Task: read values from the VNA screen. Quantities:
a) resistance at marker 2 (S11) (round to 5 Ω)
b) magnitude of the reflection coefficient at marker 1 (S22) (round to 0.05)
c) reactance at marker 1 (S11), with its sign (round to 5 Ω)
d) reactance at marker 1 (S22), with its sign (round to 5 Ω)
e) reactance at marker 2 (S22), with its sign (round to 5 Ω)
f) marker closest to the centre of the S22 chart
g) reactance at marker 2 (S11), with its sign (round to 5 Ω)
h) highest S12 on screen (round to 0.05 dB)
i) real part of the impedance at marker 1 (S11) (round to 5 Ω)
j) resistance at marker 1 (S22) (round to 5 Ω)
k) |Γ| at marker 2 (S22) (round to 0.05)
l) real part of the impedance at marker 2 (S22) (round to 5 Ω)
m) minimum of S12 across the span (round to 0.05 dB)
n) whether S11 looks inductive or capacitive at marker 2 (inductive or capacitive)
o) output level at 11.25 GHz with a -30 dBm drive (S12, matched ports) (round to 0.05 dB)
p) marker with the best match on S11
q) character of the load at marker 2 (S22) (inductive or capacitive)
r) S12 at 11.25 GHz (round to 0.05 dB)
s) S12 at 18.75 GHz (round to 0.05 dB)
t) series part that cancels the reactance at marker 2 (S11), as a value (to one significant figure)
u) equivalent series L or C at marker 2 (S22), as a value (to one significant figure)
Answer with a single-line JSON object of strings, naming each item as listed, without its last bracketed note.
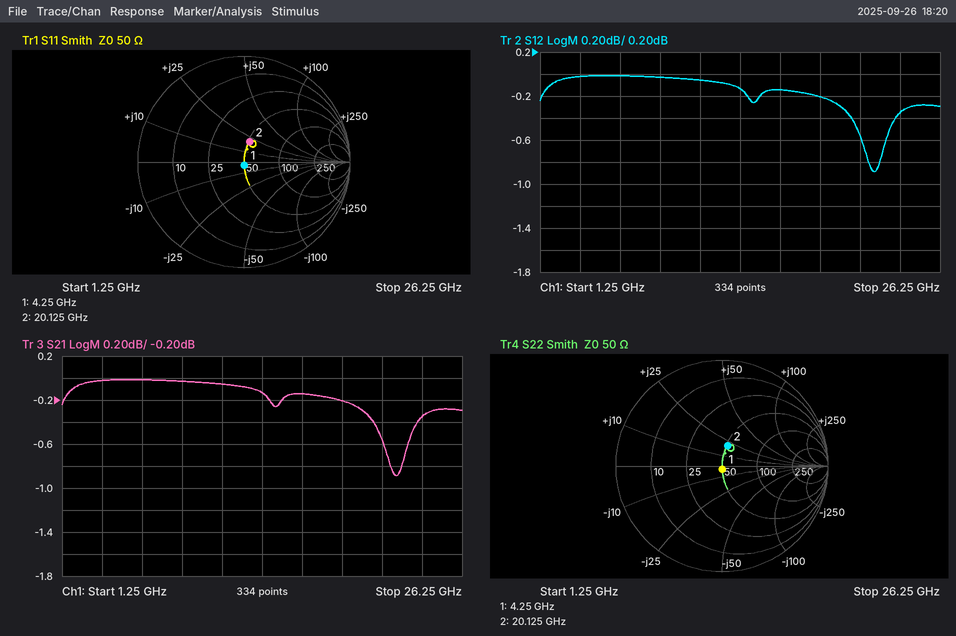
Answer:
{"resistance at marker 2 (S11)": "50 Ω", "magnitude of the reflection coefficient at marker 1 (S22)": "0.05", "reactance at marker 1 (S11), with its sign": "-5 Ω", "reactance at marker 1 (S22), with its sign": "-5 Ω", "reactance at marker 2 (S22), with its sign": "+20 Ω", "marker closest to the centre of the S22 chart": "marker 1", "reactance at marker 2 (S11), with its sign": "+20 Ω", "highest S12 on screen": "0.00 dB", "real part of the impedance at marker 1 (S11)": "50 Ω", "resistance at marker 1 (S22)": "50 Ω", "|Γ| at marker 2 (S22)": "0.20", "real part of the impedance at marker 2 (S22)": "50 Ω", "minimum of S12 across the span": "-0.90 dB", "whether S11 looks inductive or capacitive at marker 2": "inductive", "output level at 11.25 GHz with a -30 dBm drive (S12, matched ports)": "-30.05 dBm", "marker with the best match on S11": "marker 1", "character of the load at marker 2 (S22)": "inductive", "S12 at 11.25 GHz": "-0.05 dB", "S12 at 18.75 GHz": "-0.20 dB", "series part that cancels the reactance at marker 2 (S11), as a value": "400 fF", "equivalent series L or C at marker 2 (S22), as a value": "200 pH"}
